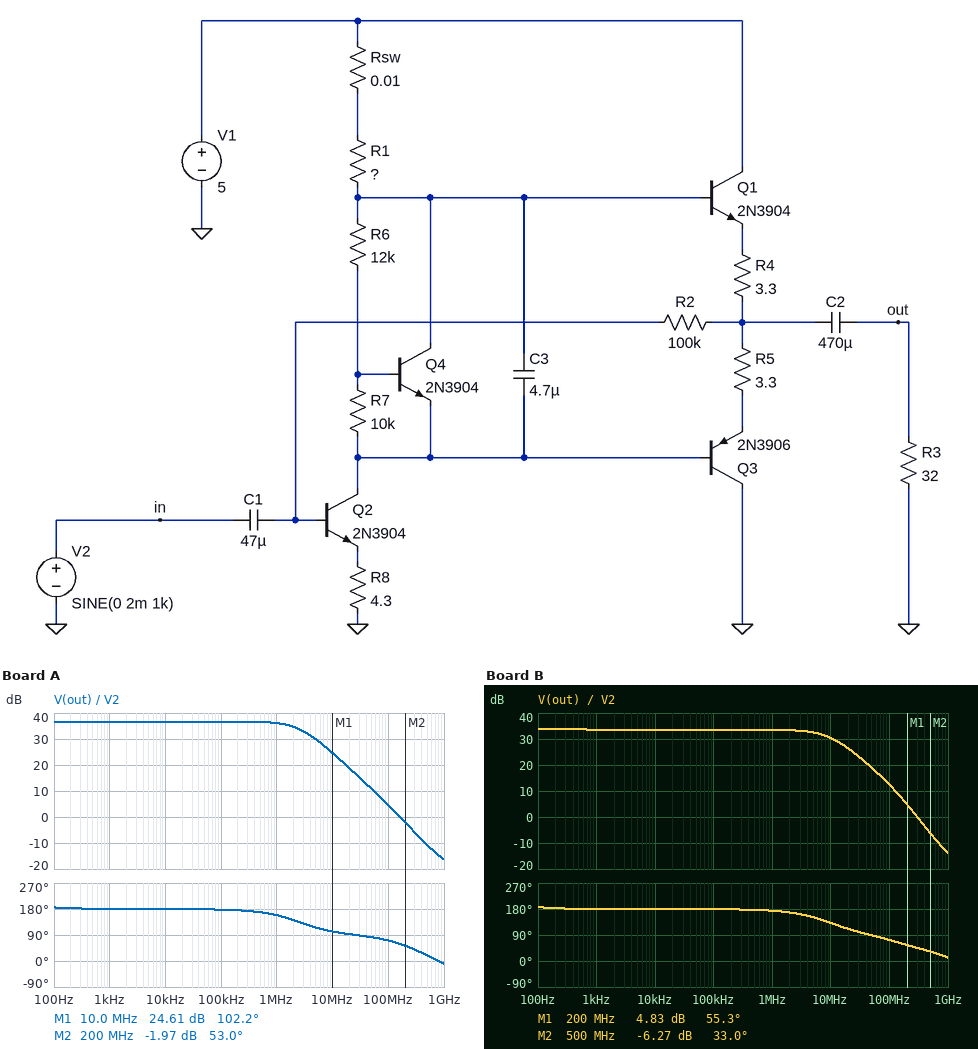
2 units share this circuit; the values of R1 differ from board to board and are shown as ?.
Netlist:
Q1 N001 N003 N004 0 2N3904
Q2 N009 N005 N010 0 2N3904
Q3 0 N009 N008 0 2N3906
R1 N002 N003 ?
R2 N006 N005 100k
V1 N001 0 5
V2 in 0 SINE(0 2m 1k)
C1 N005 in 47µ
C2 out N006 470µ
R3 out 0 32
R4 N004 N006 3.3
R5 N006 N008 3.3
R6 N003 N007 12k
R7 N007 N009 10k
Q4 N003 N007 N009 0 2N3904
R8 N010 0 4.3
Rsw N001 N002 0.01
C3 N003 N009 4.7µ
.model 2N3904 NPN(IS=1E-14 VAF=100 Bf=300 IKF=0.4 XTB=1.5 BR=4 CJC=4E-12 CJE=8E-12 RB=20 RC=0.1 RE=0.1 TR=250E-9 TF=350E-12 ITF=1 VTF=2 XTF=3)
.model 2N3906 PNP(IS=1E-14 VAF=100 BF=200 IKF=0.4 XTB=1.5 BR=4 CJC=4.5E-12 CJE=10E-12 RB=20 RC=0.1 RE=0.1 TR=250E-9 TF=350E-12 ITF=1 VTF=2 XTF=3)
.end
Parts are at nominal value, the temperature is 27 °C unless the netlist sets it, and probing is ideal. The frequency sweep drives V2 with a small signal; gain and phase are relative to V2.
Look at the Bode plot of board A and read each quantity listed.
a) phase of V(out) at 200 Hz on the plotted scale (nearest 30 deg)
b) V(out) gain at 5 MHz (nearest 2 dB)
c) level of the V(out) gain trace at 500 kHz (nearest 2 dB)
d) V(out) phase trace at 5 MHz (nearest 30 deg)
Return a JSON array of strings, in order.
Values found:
["180 deg", "30 dB", "36 dB", "120 deg"]
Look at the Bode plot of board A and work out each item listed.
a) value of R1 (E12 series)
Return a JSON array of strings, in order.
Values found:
["3.3 kΩ"]
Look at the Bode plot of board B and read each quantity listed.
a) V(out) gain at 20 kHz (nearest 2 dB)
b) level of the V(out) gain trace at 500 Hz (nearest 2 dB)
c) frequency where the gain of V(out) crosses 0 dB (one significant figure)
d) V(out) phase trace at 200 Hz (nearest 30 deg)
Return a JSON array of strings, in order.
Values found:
["34 dB", "34 dB", "300 MHz", "180 deg"]
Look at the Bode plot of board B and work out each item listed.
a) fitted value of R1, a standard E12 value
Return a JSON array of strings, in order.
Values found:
["680 Ω"]
